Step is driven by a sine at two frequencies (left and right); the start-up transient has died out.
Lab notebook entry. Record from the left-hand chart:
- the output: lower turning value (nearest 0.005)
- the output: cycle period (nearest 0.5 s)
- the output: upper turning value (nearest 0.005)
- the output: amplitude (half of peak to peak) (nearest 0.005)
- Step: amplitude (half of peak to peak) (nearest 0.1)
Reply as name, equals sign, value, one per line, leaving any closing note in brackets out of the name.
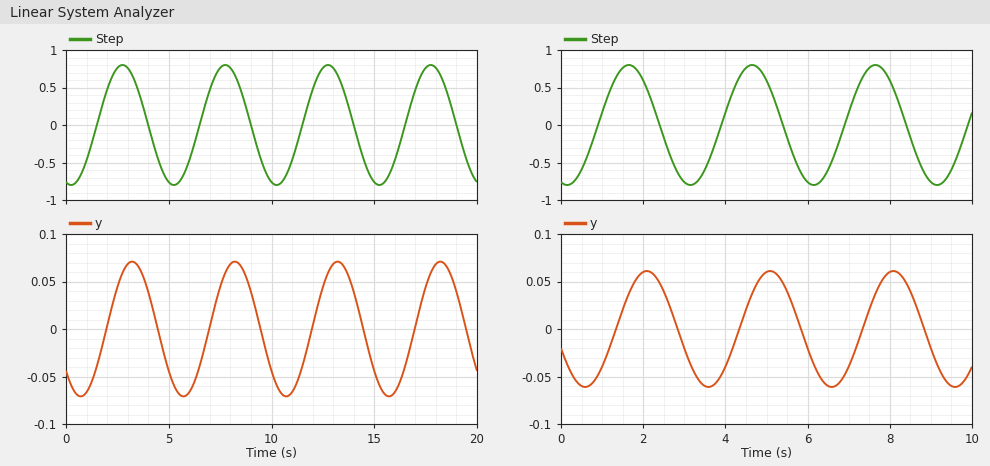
the output: lower turning value = -0.070
the output: cycle period = 5.0 s
the output: upper turning value = 0.070
the output: amplitude (half of peak to peak) = 0.070
Step: amplitude (half of peak to peak) = 0.8
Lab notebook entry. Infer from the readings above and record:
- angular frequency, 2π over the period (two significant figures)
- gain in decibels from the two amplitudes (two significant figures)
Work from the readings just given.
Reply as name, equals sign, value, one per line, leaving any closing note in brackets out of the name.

angular frequency, 2π over the period = 1.3 rad/s
gain in decibels from the two amplitudes = -21 dB
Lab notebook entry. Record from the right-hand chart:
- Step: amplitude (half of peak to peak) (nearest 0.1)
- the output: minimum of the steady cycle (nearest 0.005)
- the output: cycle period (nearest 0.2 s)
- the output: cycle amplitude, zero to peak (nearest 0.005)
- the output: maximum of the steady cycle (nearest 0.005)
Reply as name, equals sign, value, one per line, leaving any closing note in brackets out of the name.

Step: amplitude (half of peak to peak) = 0.8
the output: minimum of the steady cycle = -0.060
the output: cycle period = 3.0 s
the output: cycle amplitude, zero to peak = 0.060
the output: maximum of the steady cycle = 0.060
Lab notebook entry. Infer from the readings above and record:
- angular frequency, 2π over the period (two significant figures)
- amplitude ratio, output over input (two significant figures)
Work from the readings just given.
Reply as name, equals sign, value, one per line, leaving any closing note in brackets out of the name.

angular frequency, 2π over the period = 2.1 rad/s
amplitude ratio, output over input = 0.075
